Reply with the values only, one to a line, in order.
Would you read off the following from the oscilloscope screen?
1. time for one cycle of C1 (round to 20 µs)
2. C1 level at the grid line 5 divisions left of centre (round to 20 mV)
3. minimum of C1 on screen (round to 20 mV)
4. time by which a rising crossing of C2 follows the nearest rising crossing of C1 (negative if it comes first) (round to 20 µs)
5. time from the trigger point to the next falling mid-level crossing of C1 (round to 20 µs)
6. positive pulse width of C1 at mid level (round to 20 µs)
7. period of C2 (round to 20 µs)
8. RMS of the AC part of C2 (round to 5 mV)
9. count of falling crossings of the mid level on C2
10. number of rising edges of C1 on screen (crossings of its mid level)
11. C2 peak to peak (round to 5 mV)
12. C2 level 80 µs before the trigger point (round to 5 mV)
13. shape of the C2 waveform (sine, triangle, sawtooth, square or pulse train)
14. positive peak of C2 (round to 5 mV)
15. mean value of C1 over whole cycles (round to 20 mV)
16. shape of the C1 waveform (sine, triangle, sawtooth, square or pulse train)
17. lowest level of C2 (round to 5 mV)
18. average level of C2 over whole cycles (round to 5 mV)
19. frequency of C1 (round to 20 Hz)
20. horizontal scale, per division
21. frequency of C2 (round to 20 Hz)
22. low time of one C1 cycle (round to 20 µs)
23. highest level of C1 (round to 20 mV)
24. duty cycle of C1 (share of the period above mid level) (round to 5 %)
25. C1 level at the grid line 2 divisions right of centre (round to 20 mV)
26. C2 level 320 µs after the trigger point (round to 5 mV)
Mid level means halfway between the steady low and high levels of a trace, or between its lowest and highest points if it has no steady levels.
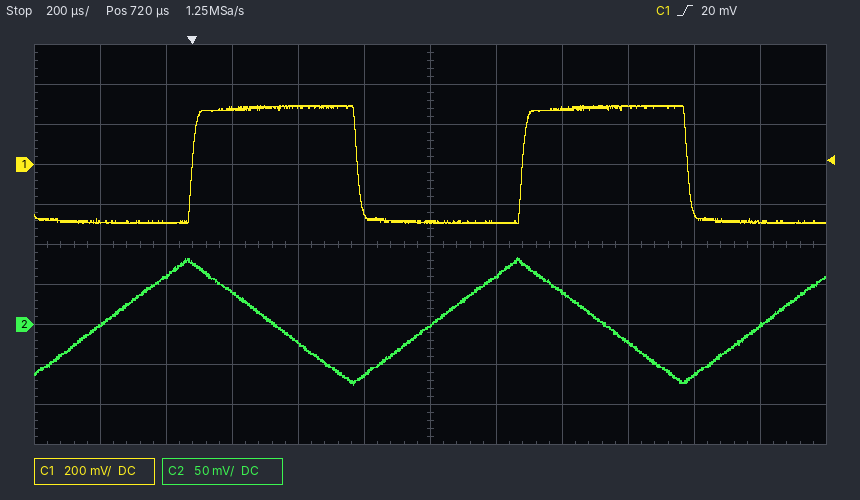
1.00 ms
-280 mV
-300 mV
-260 µs
500 µs
500 µs
1.00 ms
45 mV
2
2
160 mV
60 mV
triangle
85 mV
0 mV
square
-75 mV
5 mV
1.00 kHz
200 µs
1.00 kHz
500 µs
300 mV
50 %
280 mV
-25 mV
